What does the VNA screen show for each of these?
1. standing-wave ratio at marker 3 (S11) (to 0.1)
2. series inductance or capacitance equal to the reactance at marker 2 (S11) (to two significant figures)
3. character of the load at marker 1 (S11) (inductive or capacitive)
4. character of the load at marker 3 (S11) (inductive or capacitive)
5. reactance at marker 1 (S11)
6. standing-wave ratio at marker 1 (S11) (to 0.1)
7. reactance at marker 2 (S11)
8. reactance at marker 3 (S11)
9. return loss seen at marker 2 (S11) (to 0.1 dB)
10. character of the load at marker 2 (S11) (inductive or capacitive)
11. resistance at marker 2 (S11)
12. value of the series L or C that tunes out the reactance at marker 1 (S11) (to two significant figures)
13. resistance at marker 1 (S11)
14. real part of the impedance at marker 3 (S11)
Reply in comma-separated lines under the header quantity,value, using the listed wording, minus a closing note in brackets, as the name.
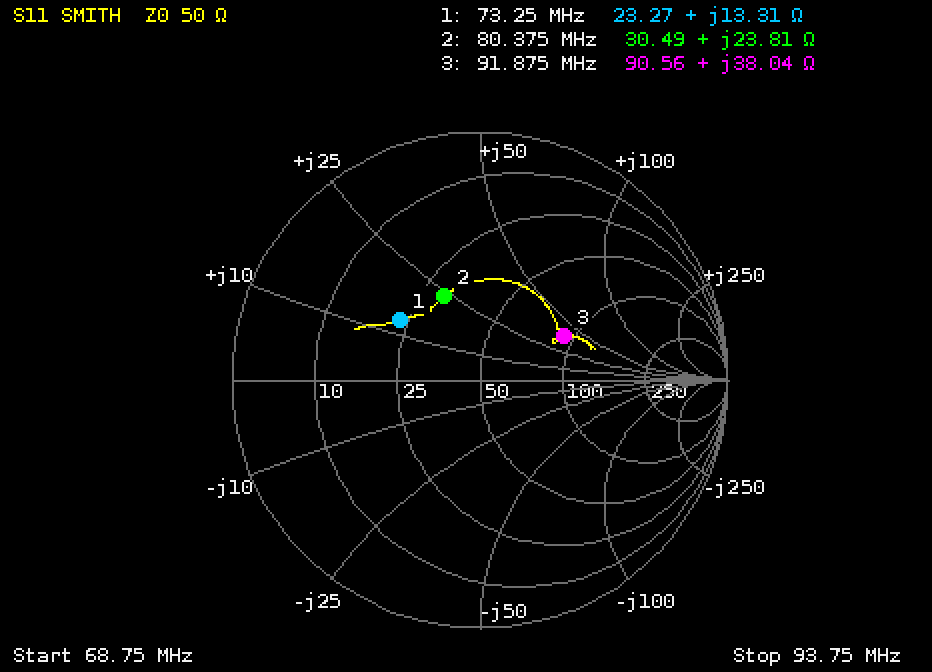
quantity,value
standing-wave ratio at marker 3 (S11),2.2
series inductance or capacitance equal to the reactance at marker 2 (S11),47 nH
character of the load at marker 1 (S11),inductive
character of the load at marker 3 (S11),inductive
reactance at marker 1,+13.31 Ω
standing-wave ratio at marker 1 (S11),2.3
reactance at marker 2,+23.81 Ω
reactance at marker 3,+38.04 Ω
return loss seen at marker 2 (S11),8.7 dB
character of the load at marker 2 (S11),inductive
resistance at marker 2,30.49 Ω
value of the series L or C that tunes out the reactance at marker 1 (S11),160 pF
resistance at marker 1,23.27 Ω
real part of the impedance at marker 3,90.56 Ω
